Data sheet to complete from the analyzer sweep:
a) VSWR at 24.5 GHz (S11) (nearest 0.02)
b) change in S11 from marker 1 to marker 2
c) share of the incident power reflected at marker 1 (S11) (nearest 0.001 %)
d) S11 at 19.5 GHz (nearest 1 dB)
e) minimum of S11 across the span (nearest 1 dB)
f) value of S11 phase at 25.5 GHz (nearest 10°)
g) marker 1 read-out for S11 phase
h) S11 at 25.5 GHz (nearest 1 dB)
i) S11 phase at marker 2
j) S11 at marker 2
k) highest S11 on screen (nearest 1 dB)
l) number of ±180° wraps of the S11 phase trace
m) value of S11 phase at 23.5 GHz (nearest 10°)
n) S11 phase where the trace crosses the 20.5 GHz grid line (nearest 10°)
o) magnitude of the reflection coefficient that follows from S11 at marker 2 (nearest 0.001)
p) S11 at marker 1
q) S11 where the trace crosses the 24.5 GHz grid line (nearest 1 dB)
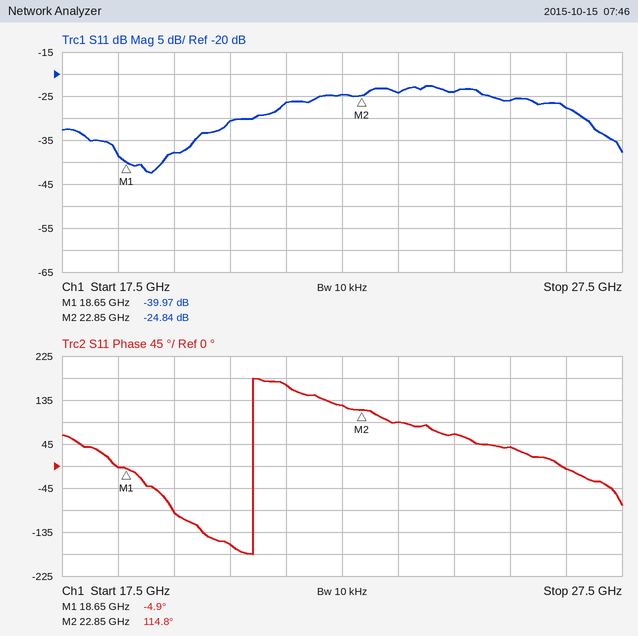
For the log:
1.14
15.13 dB
0.010 %
-38 dB
-42 dB
40°
-4.9°
-26 dB
114.8°
-24.84 dB
-23 dB
1
90°
-160°
0.057
-39.97 dB
-24 dB
